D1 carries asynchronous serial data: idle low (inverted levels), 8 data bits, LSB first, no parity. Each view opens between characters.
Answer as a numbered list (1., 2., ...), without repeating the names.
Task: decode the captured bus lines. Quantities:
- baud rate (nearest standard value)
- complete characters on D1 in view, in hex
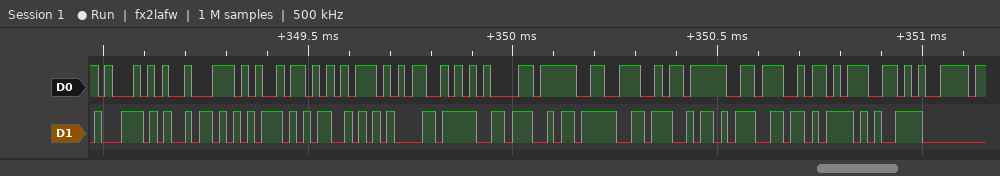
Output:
1. 57600 baud
2. 47, 4B, 45, 59, 3D, 30, 2C, 30, 2C, 31, 0A, 0D
